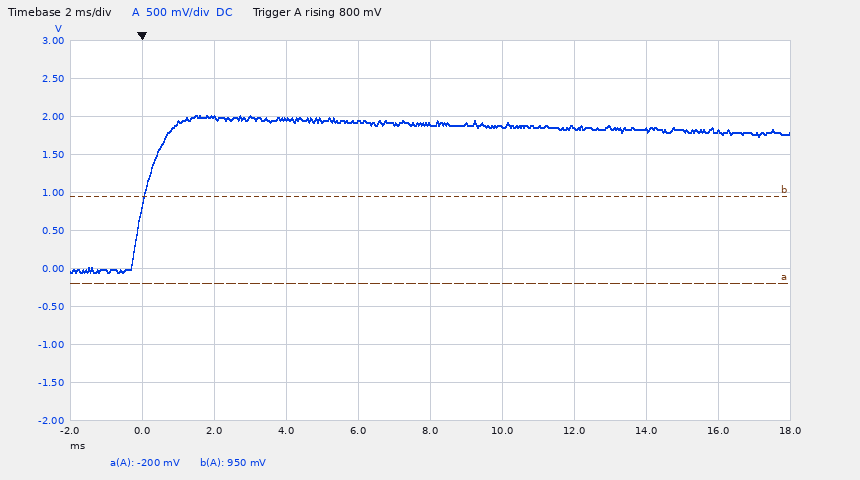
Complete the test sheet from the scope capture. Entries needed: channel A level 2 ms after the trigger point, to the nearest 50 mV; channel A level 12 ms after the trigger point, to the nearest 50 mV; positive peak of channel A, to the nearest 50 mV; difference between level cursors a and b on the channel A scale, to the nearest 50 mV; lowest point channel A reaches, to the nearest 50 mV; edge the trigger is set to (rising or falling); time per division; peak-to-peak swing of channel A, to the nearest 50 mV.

2.00 V
1.85 V
2.00 V
1.15 V
-50 mV
rising
2 ms
2.05 V
